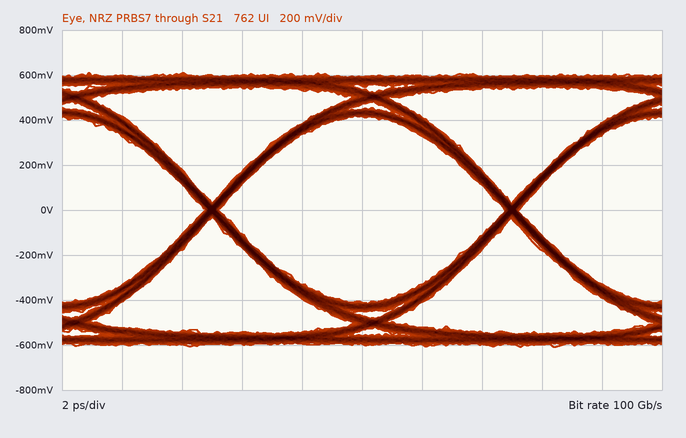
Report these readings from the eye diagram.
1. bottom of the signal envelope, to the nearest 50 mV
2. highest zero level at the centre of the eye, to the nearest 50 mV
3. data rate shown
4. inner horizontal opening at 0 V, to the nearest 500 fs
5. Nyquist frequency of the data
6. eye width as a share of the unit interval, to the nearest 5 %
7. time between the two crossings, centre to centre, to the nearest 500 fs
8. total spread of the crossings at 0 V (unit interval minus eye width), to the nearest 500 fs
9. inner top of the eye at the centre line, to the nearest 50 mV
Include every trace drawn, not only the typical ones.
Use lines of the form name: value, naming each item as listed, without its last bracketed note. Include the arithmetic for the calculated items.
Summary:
bottom of the signal envelope, to the nearest 50 mV: -600 mV
highest zero level at the centre of the eye, to the nearest 50 mV: -400 mV
data rate shown: 100 Gb/s
inner horizontal opening at 0 V, to the nearest 500 fs: 9.5 ps
Nyquist frequency of the data: 50 GHz
eye width as a share of the unit interval, to the nearest 5 %: 9.5 ps / 10.0 ps ≈ 95 %
time between the two crossings, centre to centre, to the nearest 500 fs: 10.0 ps
total spread of the crossings at 0 V (unit interval minus eye width), to the nearest 500 fs: 500 fs
inner top of the eye at the centre line, to the nearest 50 mV: 400 mV
